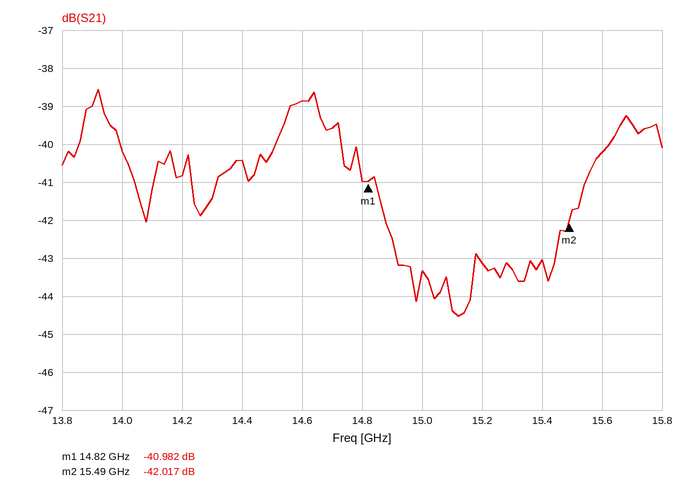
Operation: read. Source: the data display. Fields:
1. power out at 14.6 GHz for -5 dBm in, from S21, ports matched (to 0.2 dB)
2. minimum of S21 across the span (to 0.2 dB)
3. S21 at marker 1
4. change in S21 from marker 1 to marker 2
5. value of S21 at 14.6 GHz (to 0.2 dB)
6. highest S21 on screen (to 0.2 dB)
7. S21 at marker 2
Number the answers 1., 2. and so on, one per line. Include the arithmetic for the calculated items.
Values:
1. -5 dBm + (-38.8 dB) = -43.8 dBm
2. -44.6 dB
3. -40.982 dB
4. -42.017 − (-40.982) = -1.035 dB
5. -38.8 dB
6. -38.6 dB
7. -42.017 dB
